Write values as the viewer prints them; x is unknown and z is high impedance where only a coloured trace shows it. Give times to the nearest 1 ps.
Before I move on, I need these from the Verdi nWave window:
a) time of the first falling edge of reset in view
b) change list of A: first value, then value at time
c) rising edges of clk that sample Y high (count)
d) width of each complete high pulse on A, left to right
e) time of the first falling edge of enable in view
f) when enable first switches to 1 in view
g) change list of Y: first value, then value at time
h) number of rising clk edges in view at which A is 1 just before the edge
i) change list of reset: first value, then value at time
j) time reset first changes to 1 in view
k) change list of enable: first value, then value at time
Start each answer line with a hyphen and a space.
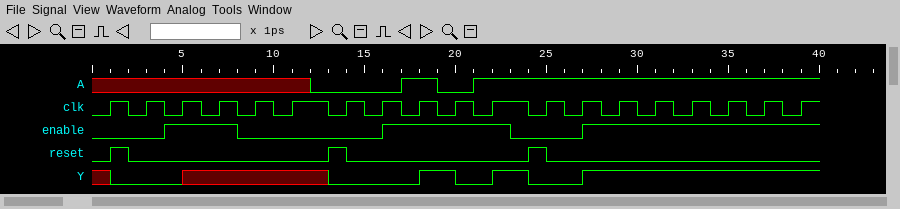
- 2 ps
- x, 0 at 12 ps, 1 at 17 ps, 0 at 19 ps, 1 at 21 ps
- 7
- 2 ps
- 8 ps
- 4 ps
- x, 0 at 1 ps, x at 5 ps, 0 at 13 ps, 1 at 18 ps, 0 at 20 ps, 1 at 22 ps, 0 at 24 ps, 1 at 27 ps
- 10
- 0, 1 at 1 ps, 0 at 2 ps, 1 at 13 ps, 0 at 14 ps, 1 at 24 ps, 0 at 25 ps
- 1 ps
- 0, 1 at 4 ps, 0 at 8 ps, 1 at 16 ps, 0 at 23 ps, 1 at 27 ps
